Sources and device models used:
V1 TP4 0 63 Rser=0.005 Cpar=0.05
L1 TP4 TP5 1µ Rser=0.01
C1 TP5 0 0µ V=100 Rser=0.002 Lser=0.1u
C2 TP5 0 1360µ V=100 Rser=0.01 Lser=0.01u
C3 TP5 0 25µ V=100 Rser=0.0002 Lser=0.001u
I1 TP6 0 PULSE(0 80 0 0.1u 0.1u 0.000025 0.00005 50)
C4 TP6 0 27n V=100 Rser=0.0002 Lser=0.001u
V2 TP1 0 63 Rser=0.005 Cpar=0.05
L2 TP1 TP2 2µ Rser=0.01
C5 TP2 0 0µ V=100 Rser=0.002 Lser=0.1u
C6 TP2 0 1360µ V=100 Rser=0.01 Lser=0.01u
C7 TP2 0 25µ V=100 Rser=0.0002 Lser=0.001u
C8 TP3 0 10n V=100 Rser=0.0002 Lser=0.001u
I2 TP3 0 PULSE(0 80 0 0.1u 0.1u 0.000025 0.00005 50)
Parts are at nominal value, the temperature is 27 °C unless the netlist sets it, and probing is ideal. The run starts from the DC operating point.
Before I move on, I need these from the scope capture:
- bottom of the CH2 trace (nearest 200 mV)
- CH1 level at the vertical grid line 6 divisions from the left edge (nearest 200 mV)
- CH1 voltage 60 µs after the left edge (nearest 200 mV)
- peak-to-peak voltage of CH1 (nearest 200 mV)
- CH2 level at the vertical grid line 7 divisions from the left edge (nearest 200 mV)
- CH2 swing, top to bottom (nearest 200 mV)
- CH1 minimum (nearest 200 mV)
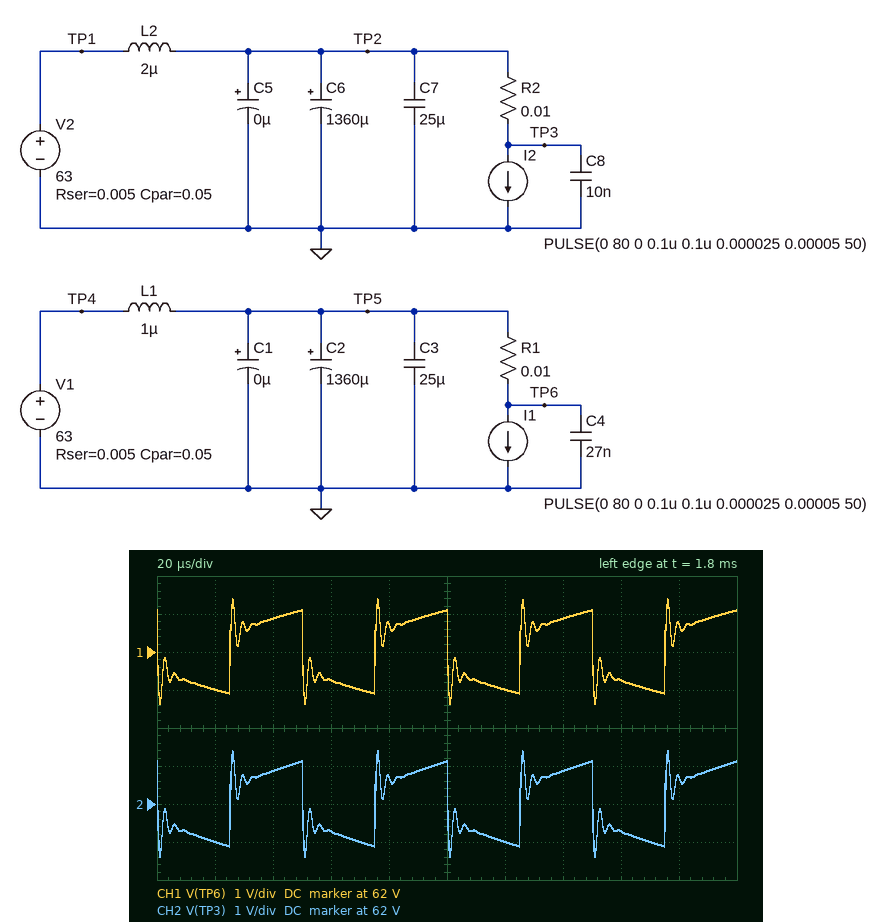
60.6 V
61.0 V
61.2 V
2.8 V
62.8 V
2.8 V
60.6 V
